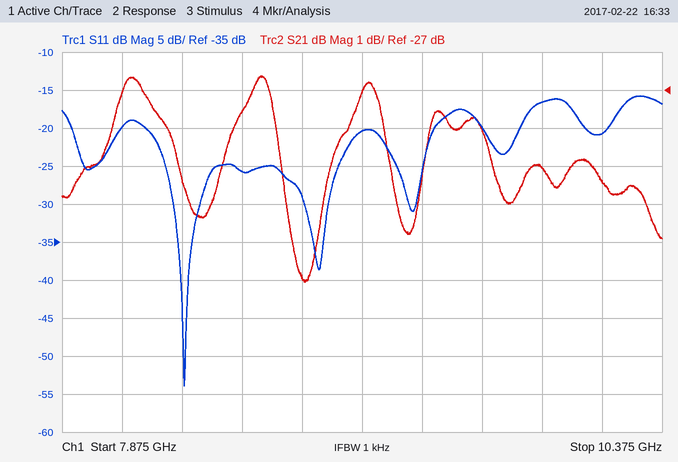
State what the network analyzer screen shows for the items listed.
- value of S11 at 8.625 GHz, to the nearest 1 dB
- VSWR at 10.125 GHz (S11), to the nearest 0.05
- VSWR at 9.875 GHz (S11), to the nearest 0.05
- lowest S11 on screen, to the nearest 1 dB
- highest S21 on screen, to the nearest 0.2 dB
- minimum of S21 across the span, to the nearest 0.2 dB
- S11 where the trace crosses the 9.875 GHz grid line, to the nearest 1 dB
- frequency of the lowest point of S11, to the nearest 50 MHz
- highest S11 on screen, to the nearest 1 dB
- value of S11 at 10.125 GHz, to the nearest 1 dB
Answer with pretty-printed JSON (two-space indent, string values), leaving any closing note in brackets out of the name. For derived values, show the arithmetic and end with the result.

{
  "value of S11 at 8.625 GHz, to the nearest 1 dB": "-26 dB",
  "VSWR at 10.125 GHz (S11), to the nearest 0.05": "|Γ| = 10^(-21/20) = 0.0891; VSWR = (1 + 0.0891)/(1 − 0.0891) ≈ 1.20",
  "VSWR at 9.875 GHz (S11), to the nearest 0.05": "|Γ| = 10^(-17/20) = 0.1413; VSWR = (1 + 0.1413)/(1 − 0.1413) ≈ 1.33, so 1.35 to the nearest 0.05",
  "lowest S11 on screen, to the nearest 1 dB": "-54 dB",
  "highest S21 on screen, to the nearest 0.2 dB": "-26.6 dB",
  "minimum of S21 across the span, to the nearest 0.2 dB": "-32.0 dB",
  "S11 where the trace crosses the 9.875 GHz grid line, to the nearest 1 dB": "-17 dB",
  "frequency of the lowest point of S11, to the nearest 50 MHz": "8.40 GHz",
  "highest S11 on screen, to the nearest 1 dB": "-16 dB",
  "value of S11 at 10.125 GHz, to the nearest 1 dB": "-21 dB"
}
